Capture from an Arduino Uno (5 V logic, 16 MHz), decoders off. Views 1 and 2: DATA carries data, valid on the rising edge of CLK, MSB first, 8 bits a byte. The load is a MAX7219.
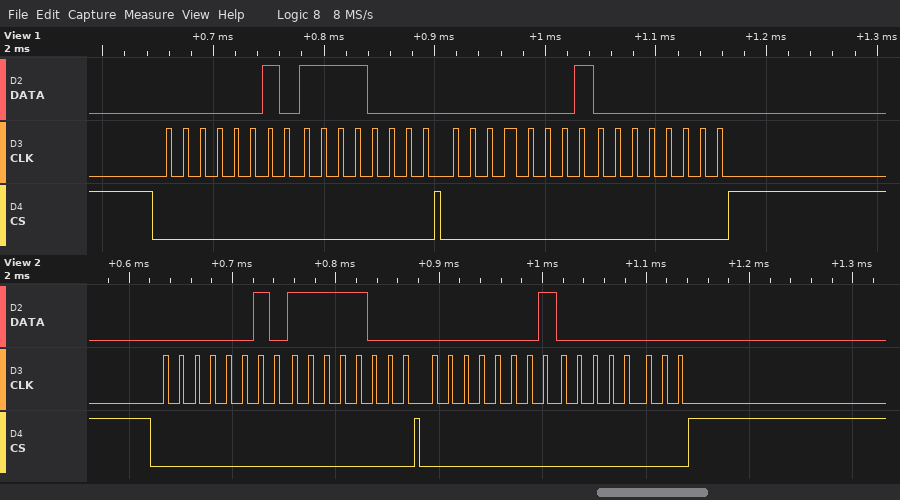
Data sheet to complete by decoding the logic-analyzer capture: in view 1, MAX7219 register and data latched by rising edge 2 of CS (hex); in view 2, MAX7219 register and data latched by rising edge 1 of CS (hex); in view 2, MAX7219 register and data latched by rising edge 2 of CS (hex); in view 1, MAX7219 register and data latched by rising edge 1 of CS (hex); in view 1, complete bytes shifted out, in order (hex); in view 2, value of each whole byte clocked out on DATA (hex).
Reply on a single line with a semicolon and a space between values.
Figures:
register 0x1, data 0x00; register 0x2, data 0xF8; register 0x1, data 0x00; register 0x2, data 0xF0; 02 F0 01 00; 0x02 0xF8 0x01 0x00
